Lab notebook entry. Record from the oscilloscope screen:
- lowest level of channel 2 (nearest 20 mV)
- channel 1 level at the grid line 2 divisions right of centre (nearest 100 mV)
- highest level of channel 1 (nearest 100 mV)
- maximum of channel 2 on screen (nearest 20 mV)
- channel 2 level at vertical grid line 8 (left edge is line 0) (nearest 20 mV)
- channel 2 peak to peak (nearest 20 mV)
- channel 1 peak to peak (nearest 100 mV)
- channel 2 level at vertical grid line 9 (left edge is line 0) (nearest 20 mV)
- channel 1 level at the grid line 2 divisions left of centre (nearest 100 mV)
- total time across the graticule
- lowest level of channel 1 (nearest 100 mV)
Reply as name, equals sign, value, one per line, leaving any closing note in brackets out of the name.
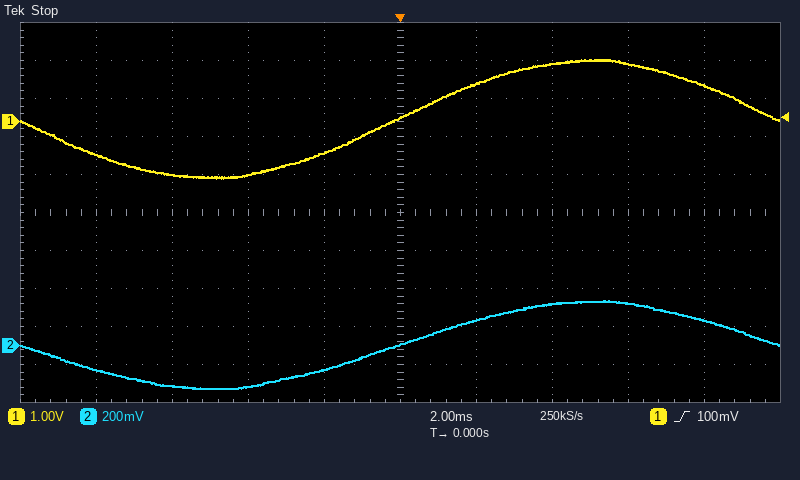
lowest level of channel 2 = -220 mV
channel 1 level at the grid line 2 divisions right of centre = 1.5 V
highest level of channel 1 = 1.6 V
maximum of channel 2 on screen = 240 mV
channel 2 level at vertical grid line 8 (left edge is line 0) = 220 mV
channel 2 peak to peak = 460 mV
channel 1 peak to peak = 3.1 V
channel 2 level at vertical grid line 9 (left edge is line 0) = 140 mV
channel 1 level at the grid line 2 divisions left of centre = -1.4 V
total time across the graticule = 20 ms
lowest level of channel 1 = -1.5 V
